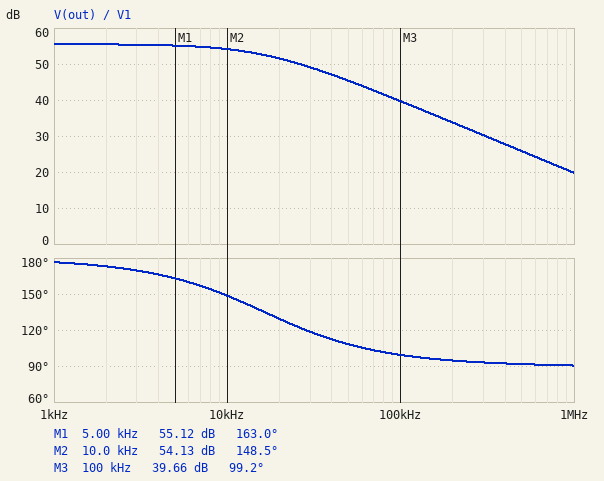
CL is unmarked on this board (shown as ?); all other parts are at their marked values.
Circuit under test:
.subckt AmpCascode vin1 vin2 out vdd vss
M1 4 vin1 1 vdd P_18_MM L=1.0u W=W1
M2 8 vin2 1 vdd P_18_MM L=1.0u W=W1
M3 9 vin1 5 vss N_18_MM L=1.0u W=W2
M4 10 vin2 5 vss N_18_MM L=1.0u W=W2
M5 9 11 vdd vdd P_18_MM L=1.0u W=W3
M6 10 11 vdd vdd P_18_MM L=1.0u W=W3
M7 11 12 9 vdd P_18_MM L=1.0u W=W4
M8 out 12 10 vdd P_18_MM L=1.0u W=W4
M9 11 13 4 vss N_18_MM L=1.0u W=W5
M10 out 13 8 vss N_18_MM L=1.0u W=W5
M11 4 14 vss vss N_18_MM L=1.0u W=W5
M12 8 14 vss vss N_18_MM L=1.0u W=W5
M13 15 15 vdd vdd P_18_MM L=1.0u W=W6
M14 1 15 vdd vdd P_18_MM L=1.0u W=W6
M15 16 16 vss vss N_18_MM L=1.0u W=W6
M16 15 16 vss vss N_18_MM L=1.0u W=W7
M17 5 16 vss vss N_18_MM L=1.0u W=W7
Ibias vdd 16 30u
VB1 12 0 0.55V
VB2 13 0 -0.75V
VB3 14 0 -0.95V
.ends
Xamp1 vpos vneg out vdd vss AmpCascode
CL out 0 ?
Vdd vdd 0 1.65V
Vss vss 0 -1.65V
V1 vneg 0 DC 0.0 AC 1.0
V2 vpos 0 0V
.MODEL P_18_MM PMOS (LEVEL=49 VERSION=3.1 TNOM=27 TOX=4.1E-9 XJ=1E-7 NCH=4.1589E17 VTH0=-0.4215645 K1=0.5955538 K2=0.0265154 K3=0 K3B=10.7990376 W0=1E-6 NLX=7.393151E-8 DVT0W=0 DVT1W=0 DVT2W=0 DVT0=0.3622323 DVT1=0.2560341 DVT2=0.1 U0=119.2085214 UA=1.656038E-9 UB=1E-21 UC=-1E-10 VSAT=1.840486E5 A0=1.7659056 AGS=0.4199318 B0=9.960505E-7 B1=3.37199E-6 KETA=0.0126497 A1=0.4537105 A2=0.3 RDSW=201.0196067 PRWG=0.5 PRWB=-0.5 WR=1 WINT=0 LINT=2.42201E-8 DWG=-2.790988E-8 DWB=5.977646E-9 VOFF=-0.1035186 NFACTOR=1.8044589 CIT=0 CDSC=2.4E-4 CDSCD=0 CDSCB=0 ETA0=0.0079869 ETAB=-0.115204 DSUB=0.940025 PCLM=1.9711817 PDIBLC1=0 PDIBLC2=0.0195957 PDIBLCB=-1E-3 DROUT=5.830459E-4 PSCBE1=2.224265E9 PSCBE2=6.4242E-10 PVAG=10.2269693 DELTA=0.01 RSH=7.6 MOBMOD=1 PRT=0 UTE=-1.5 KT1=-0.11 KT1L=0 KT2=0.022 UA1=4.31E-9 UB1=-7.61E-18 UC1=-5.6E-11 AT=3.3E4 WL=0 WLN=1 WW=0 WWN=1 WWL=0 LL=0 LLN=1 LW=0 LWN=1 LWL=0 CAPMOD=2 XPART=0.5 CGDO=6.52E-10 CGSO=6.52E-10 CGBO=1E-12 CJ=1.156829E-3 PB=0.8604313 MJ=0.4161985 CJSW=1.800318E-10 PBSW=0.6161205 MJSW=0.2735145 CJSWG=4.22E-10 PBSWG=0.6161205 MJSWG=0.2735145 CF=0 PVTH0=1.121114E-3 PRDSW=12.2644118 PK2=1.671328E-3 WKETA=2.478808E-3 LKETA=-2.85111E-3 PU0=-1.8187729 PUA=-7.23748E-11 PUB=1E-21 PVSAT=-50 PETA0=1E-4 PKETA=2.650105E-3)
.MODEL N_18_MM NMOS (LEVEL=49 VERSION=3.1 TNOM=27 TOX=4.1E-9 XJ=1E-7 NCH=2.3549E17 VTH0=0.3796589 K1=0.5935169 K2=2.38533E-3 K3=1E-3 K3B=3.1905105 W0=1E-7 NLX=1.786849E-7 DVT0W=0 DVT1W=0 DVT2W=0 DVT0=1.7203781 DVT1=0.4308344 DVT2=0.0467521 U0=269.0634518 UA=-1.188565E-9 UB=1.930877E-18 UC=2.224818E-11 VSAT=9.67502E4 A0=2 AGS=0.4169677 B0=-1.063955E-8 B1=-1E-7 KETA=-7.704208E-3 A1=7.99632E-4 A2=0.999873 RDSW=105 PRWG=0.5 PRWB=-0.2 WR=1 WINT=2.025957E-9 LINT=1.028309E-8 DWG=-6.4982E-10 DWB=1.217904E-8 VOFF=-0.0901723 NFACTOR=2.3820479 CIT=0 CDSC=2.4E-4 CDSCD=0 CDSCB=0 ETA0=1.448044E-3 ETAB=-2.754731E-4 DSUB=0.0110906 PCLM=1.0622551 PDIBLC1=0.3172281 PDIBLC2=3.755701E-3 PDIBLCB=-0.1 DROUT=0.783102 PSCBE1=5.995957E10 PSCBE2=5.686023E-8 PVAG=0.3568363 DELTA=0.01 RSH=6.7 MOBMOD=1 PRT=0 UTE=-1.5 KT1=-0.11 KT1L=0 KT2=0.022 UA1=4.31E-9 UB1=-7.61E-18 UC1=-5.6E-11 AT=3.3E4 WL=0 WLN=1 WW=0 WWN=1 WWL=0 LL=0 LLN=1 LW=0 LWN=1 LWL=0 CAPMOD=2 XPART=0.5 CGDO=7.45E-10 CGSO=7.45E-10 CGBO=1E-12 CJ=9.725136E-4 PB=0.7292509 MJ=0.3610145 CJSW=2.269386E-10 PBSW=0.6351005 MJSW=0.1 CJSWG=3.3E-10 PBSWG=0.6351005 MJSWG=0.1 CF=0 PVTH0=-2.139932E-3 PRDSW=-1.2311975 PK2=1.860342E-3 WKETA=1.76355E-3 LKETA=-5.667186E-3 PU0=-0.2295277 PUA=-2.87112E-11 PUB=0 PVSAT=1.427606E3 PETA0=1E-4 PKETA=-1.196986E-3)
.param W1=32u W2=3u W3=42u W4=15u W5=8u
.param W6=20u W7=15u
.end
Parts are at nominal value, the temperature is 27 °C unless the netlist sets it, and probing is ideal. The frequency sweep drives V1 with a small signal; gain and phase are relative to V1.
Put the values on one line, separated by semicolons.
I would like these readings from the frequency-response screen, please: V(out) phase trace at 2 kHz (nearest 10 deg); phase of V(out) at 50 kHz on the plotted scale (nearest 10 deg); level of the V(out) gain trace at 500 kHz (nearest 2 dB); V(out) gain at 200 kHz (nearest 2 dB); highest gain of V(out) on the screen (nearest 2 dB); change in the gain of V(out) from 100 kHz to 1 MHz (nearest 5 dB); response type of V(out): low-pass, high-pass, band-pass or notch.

170 deg; 110 deg; 26 dB; 34 dB; 56 dB; -20 dB; low-pass
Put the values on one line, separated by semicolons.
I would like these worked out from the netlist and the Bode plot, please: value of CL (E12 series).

4.7 pF
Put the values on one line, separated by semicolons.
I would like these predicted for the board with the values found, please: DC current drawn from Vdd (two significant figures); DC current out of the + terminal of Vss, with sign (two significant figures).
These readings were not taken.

200 µA; -200 µA
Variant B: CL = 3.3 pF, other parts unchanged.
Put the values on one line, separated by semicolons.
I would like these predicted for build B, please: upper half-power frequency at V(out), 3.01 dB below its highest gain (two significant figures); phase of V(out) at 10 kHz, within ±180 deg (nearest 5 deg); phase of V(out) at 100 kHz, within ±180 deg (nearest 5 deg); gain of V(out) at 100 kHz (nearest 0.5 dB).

23 kHz; 155 deg; 105 deg; 42.5 dB
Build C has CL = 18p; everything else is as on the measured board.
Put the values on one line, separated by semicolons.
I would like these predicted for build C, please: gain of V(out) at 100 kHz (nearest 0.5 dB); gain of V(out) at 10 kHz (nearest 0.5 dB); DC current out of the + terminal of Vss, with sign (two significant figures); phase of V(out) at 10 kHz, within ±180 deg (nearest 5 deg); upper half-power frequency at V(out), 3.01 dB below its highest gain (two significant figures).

28.0 dB; 47.5 dB; -200 µA; 115 deg; 4.3 kHz
